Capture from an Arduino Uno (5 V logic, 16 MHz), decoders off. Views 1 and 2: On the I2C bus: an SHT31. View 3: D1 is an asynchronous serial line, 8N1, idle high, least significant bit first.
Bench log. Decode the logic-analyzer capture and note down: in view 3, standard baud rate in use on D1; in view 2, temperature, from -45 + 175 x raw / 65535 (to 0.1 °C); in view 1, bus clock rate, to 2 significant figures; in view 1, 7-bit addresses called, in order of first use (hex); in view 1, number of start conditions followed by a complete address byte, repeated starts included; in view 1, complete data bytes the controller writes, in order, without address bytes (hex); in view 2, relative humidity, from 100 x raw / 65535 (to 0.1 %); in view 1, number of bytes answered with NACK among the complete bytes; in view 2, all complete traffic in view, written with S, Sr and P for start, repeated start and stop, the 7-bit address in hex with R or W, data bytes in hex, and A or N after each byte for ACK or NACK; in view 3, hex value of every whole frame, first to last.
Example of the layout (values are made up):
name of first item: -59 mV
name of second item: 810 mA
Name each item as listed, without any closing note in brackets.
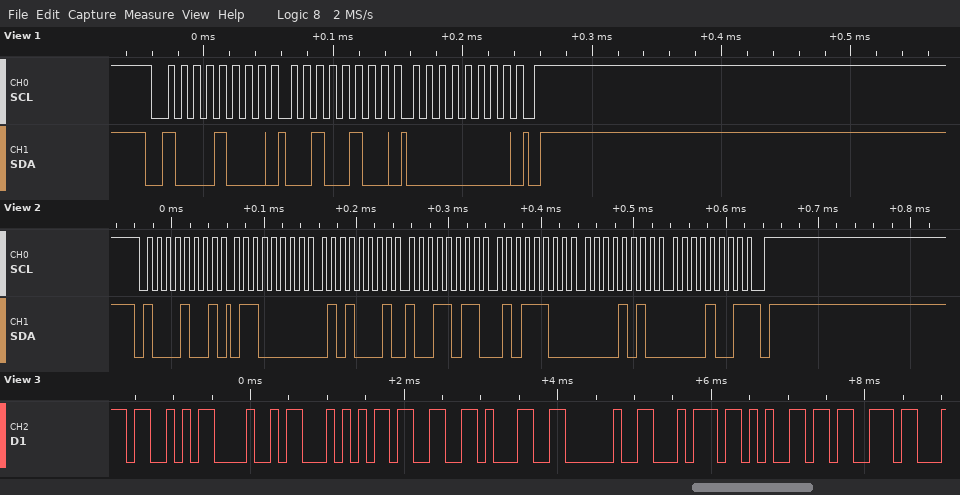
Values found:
in view 3, standard baud rate in use on D1: 9600 baud
in view 2, temperature, from -45 + 175 x raw / 65535: 20.8 °C
in view 1, bus clock rate, to 2 significant figures: 100 kHz
in view 1, 7-bit addresses called, in order of first use: 0x44
in view 1, number of start conditions followed by a complete address byte, repeated starts included: 1
in view 1, complete data bytes the controller writes, in order, without address bytes: 24 00
in view 2, relative humidity, from 100 x raw / 65535: 36.0 %
in view 1, number of bytes answered with NACK among the complete bytes: 0
in view 2, all complete traffic in view, written with S, Sr and P for start, repeated start and stop, the 7-bit address in hex with R or W, data bytes in hex, and A or N after each byte for ACK or NACK: S 44R A 60 A 51 A 9B A 5C A 0A A 09 N P
in view 3, hex value of every whole frame, first to last: 53 48 54 33 31 20 74 65 73
